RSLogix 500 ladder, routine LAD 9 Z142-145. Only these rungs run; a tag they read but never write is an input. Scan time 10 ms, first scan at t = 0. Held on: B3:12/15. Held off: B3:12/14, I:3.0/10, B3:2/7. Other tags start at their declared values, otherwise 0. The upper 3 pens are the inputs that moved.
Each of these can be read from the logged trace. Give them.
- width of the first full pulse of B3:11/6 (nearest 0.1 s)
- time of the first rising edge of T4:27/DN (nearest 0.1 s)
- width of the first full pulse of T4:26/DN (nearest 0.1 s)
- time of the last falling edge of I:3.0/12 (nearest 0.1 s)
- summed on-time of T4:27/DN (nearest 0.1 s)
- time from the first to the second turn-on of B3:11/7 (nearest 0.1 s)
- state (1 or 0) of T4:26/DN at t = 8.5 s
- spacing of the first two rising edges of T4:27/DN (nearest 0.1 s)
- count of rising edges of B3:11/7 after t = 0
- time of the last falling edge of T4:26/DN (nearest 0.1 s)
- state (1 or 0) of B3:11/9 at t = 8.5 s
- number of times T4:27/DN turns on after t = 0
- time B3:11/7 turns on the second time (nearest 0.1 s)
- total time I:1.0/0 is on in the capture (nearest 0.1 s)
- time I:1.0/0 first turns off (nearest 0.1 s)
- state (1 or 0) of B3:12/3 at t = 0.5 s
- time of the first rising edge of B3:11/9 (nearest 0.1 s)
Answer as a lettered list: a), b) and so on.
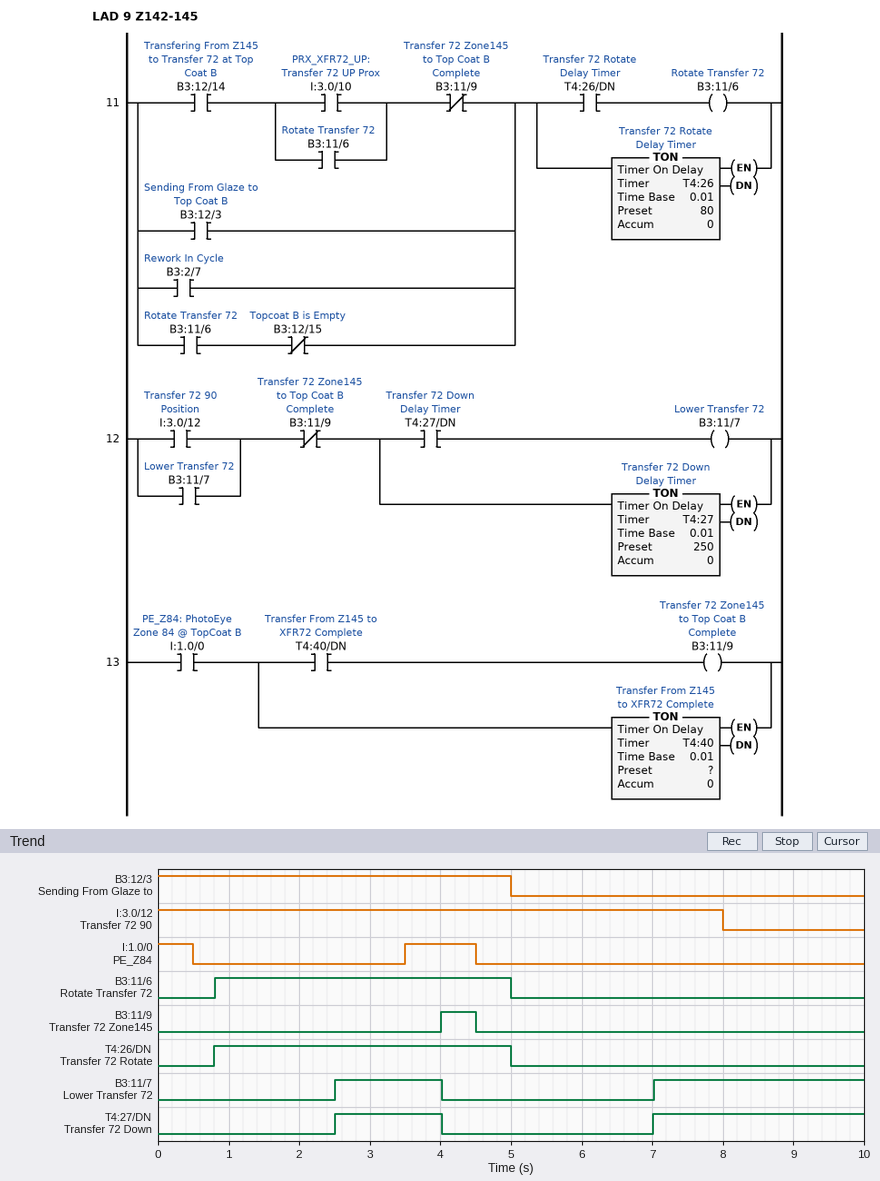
a) 4.2 s
b) 2.5 s
c) 4.2 s
d) 8.0 s
e) 4.5 s
f) 4.5 s
g) 0
h) 4.5 s
i) 2
j) 5.0 s
k) 0
l) 2
m) 7.0 s
n) 1.5 s
o) 0.5 s
p) 1
q) 4.0 s
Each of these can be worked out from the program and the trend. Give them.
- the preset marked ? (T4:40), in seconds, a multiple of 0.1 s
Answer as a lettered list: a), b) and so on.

a) 0.5 s
